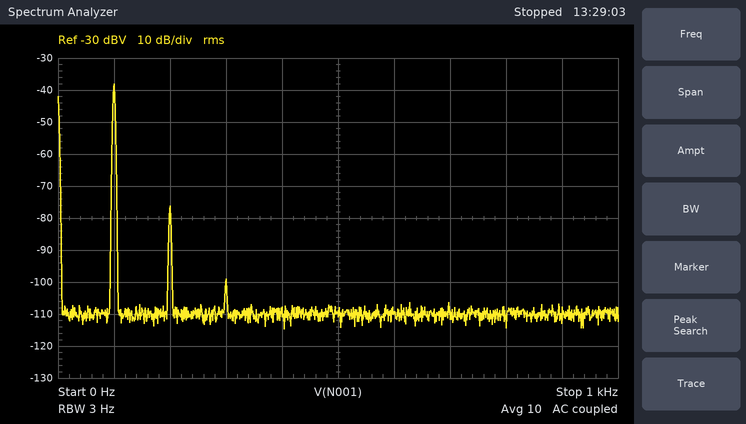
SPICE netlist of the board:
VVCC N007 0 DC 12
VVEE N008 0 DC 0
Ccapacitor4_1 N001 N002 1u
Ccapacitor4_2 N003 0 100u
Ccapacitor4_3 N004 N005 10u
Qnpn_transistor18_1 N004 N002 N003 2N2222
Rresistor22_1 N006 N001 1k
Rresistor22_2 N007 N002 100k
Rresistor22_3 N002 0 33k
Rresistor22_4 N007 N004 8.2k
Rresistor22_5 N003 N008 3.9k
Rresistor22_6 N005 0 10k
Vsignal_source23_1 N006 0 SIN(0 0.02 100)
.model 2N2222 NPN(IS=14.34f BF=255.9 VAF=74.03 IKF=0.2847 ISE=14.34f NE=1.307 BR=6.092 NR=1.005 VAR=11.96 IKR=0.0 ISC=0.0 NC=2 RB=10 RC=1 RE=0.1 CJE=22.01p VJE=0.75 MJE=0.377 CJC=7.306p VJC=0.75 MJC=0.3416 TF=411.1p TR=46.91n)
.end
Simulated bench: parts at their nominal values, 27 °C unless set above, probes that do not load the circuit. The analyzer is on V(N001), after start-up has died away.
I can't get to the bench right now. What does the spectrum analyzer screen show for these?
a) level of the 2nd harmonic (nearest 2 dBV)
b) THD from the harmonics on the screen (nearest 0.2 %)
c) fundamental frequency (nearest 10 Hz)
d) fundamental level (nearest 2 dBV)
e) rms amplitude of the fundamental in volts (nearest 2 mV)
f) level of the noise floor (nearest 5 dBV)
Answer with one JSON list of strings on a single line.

["-76 dBV", "1.2 %", "100 Hz", "-38 dBV", "12 mV", "-110 dBV"]
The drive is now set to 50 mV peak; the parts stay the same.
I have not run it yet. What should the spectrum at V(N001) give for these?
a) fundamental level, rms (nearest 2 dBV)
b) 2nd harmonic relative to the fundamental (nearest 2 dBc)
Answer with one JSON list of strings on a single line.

["-30 dBV", "-32 dBc"]
